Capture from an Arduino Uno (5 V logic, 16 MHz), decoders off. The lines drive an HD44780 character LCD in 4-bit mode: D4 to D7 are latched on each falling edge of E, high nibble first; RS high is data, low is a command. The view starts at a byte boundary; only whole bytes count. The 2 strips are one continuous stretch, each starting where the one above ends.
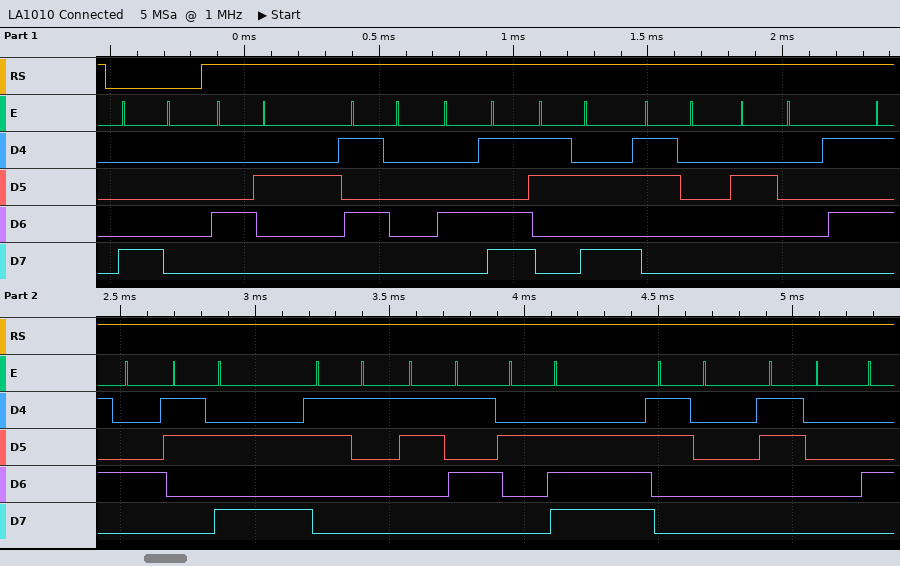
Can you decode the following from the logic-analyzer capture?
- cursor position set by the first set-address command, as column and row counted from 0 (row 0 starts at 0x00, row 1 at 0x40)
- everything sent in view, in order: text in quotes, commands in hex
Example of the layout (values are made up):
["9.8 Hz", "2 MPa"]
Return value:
["column 0, row 0", "0x80 \"BPM:0 T:15.00\""]
